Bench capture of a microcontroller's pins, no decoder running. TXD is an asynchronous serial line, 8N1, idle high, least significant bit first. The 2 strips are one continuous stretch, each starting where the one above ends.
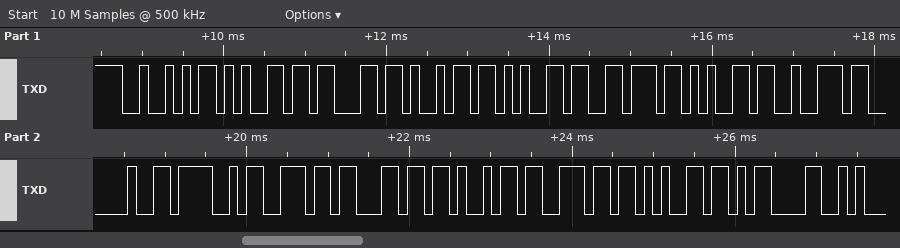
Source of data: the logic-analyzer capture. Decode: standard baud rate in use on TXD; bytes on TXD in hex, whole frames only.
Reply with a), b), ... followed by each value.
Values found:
a) 9600 baud
b) 52 65 63 69 65 76 65 72 20 4F 6E 6C 69 6E 65 0D
